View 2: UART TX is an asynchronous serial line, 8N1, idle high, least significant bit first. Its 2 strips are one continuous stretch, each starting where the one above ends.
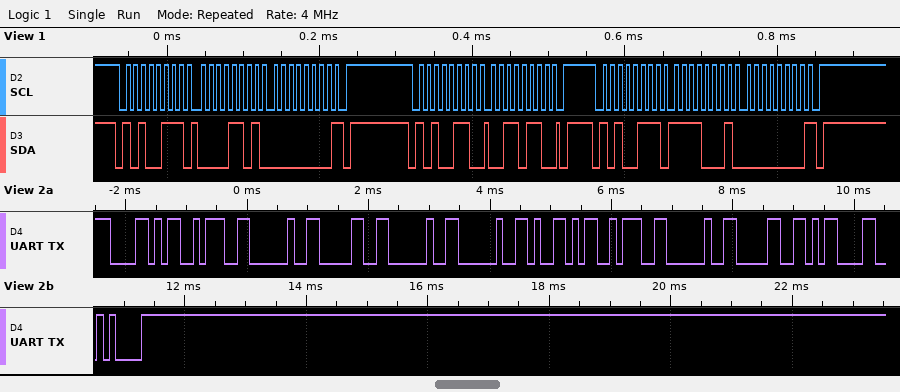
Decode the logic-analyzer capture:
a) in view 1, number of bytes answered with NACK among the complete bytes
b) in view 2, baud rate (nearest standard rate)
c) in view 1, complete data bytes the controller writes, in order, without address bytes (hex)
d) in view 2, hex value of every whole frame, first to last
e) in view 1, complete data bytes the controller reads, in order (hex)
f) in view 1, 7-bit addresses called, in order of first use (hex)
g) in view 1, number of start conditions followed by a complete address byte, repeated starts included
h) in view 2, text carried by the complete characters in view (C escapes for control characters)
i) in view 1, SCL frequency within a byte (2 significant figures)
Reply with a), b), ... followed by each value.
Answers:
a) 2
b) 9600 baud
c) 36
d) 58 3A 20 30 20 20 59 3A 20 30 0D 0A
e) 0D 00 F1 00
f) 0x53
g) 3
h) "X: 0  Y: 0\r\n"
i) 100 kHz
